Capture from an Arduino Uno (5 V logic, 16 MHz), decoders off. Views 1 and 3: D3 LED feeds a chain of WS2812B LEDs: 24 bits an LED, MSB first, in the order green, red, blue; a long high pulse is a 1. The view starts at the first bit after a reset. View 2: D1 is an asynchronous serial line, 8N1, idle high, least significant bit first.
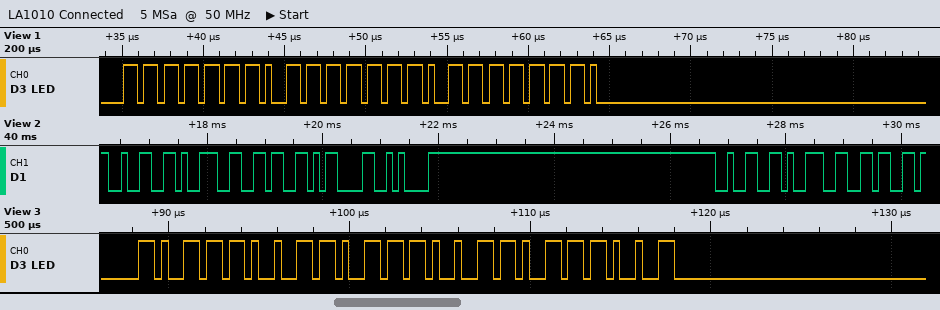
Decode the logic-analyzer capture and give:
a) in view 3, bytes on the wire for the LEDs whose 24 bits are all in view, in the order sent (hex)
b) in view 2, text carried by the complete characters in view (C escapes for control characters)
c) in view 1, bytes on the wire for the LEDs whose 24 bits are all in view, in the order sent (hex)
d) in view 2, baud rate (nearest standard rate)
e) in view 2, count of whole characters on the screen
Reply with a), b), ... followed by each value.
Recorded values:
a) B9 B9 B9
b) "296\r\n296"
c) FE FE FE
d) 9600 baud
e) 8
